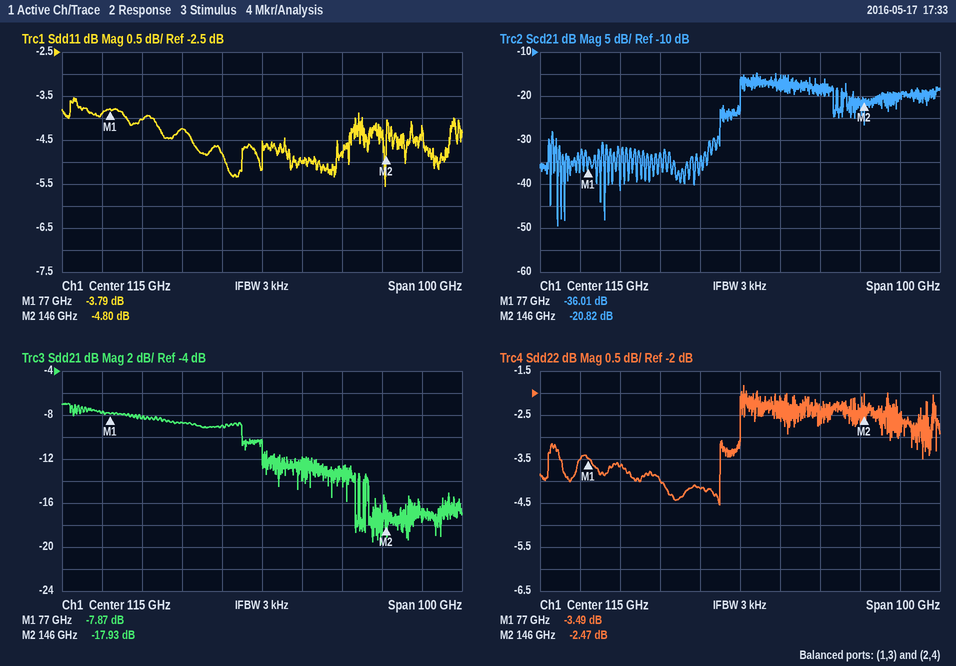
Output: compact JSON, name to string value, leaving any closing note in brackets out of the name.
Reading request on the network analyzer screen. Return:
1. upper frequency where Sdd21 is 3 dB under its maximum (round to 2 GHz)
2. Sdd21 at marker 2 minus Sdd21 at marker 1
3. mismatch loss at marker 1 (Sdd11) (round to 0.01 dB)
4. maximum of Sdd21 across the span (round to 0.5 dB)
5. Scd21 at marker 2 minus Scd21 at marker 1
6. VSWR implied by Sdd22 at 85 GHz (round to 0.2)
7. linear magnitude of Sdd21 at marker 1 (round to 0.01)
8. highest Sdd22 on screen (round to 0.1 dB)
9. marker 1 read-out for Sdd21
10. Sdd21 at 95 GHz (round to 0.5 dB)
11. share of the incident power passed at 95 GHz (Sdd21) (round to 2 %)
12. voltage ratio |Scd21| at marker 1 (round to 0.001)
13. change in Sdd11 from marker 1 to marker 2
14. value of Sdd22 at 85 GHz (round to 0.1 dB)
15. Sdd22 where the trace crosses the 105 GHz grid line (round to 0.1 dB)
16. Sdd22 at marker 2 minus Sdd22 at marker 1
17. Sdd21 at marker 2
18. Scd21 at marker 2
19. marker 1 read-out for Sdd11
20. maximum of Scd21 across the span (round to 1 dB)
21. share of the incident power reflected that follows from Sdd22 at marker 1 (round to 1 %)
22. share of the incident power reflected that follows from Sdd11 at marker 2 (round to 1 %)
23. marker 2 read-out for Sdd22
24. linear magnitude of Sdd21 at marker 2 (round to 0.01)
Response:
{"upper frequency where Sdd21 is 3 dB under its maximum": "110 GHz", "Sdd21 at marker 2 minus Sdd21 at marker 1": "-10.06 dB", "mismatch loss at marker 1 (Sdd11)": "2.35 dB", "maximum of Sdd21 across the span": "-7.0 dB", "Scd21 at marker 2 minus Scd21 at marker 1": "15.19 dB", "VSWR implied by Sdd22 at 85 GHz": "4.8", "linear magnitude of Sdd21 at marker 1": "0.40", "highest Sdd22 on screen": "-1.8 dB", "marker 1 read-out for Sdd21": "-7.87 dB", "Sdd21 at 95 GHz": "-8.5 dB", "share of the incident power passed at 95 GHz (Sdd21)": "14 %", "voltage ratio |Scd21| at marker 1": "0.016", "change in Sdd11 from marker 1 to marker 2": "-1.01 dB", "value of Sdd22 at 85 GHz": "-3.7 dB", "Sdd22 where the trace crosses the 105 GHz grid line": "-4.2 dB", "Sdd22 at marker 2 minus Sdd22 at marker 1": "1.02 dB", "Sdd21 at marker 2": "-17.93 dB", "Scd21 at marker 2": "-20.82 dB", "marker 1 read-out for Sdd11": "-3.79 dB", "maximum of Scd21 across the span": "-15 dB", "share of the incident power reflected that follows from Sdd22 at marker 1": "45 %", "share of the incident power reflected that follows from Sdd11 at marker 2": "33 %", "marker 2 read-out for Sdd22": "-2.47 dB", "linear magnitude of Sdd21 at marker 2": "0.13"}
